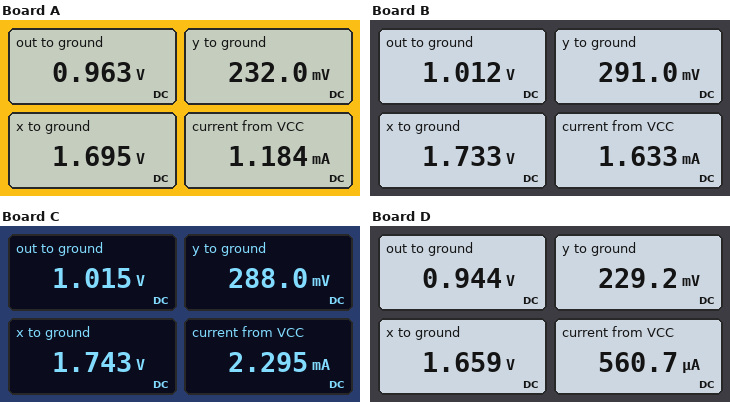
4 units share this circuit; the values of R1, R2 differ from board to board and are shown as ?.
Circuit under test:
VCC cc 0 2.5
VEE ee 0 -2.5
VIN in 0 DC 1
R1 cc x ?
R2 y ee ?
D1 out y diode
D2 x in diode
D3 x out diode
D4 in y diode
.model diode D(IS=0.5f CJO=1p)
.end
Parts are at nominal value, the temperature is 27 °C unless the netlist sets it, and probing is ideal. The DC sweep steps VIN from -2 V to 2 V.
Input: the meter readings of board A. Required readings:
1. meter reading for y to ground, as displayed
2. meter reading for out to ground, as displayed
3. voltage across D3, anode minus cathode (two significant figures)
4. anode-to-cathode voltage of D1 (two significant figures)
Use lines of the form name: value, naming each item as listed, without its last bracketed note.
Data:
meter reading for y to ground, as displayed: 232.0 mV
meter reading for out to ground, as displayed: 0.963 V
voltage across D3, anode minus cathode: 730 mV
anode-to-cathode voltage of D1: 730 mV
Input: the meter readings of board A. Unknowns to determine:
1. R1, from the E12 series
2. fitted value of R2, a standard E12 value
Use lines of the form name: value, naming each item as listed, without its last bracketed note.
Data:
R1, from the E12 series: 680 Ω
fitted value of R2, a standard E12 value: 560 Ω
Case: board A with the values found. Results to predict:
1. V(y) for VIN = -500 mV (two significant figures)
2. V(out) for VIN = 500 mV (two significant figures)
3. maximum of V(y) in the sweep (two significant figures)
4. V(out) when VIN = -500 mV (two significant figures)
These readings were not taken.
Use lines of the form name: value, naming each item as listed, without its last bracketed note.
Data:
V(y) for VIN = -500 mV: -1.2 V
V(out) for VIN = 500 mV: 480 mV
maximum of V(y) in the sweep: 1.2 V
V(out) when VIN = -500 mV: -490 mV
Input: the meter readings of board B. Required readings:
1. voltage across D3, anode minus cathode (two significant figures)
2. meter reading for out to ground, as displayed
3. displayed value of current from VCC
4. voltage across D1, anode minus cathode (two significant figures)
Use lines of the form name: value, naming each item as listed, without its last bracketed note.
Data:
voltage across D3, anode minus cathode: 720 mV
meter reading for out to ground, as displayed: 1.012 V
displayed value of current from VCC: 1.633 mA
voltage across D1, anode minus cathode: 720 mV
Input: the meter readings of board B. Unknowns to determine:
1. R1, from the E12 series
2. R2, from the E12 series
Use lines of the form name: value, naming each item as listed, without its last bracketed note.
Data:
R1, from the E12 series: 470 Ω
R2, from the E12 series: 2.7 kΩ
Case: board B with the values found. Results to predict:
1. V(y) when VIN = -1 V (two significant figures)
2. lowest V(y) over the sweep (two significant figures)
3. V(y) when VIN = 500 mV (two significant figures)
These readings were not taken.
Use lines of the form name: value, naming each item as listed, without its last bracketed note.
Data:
V(y) when VIN = -1 V: -1.6 V
lowest V(y) over the sweep: -2.5 V
V(y) when VIN = 500 mV: -190 mV
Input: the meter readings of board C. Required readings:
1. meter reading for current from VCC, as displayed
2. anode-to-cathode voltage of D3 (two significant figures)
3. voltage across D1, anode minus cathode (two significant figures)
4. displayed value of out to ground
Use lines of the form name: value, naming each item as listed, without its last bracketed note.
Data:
meter reading for current from VCC, as displayed: 2.295 mA
anode-to-cathode voltage of D3: 730 mV
voltage across D1, anode minus cathode: 730 mV
displayed value of out to ground: 1.015 V
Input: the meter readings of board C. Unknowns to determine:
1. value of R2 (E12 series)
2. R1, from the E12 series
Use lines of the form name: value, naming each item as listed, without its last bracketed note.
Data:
value of R2: 2.2 kΩ
R1, from the E12 series: 330 Ω
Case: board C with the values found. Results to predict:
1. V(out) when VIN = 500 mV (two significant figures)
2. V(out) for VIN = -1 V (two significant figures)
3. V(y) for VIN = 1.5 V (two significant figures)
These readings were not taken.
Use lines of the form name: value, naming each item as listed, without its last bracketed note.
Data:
V(out) when VIN = 500 mV: 530 mV
V(out) for VIN = -1 V: -920 mV
V(y) for VIN = 1.5 V: 770 mV
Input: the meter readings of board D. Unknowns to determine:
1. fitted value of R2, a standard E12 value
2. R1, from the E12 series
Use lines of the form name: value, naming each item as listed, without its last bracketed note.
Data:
fitted value of R2, a standard E12 value: 560 Ω
R1, from the E12 series: 1.5 kΩ
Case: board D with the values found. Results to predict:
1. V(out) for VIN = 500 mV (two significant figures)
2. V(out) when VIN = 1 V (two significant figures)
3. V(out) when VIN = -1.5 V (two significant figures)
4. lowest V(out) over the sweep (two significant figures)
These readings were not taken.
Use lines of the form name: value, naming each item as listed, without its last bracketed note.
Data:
V(out) for VIN = 500 mV: 460 mV
V(out) when VIN = 1 V: 940 mV
V(out) when VIN = -1.5 V: -1.5 V
lowest V(out) over the sweep: -1.9 V
